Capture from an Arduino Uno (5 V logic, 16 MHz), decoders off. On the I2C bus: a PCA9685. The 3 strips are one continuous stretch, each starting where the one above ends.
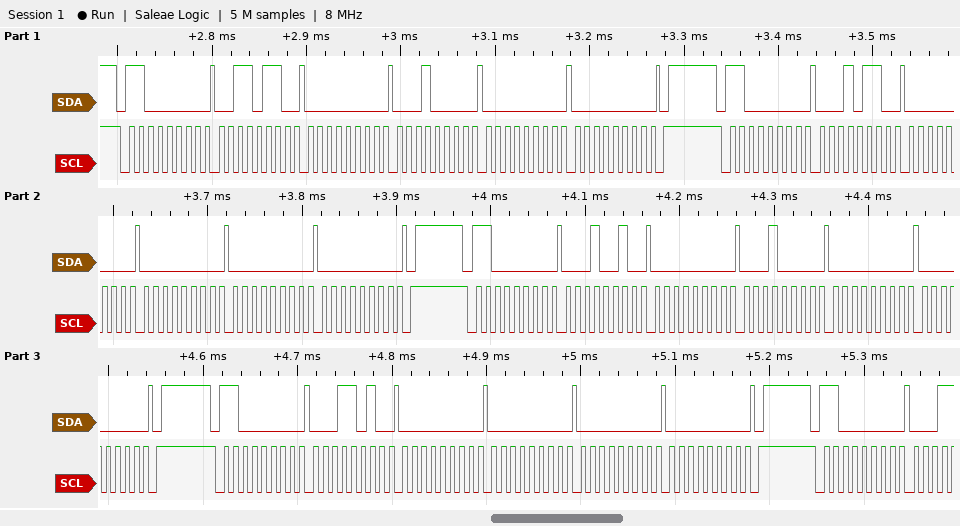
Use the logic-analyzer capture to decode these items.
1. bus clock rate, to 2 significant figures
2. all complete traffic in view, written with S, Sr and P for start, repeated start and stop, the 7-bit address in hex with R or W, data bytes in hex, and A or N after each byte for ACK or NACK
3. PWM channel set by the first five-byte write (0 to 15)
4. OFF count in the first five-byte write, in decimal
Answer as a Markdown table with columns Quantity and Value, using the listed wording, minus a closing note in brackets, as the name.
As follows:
| Quantity | Value |
|---|---|
| bus clock rate, to 2 significant figures | 100 kHz |
| all complete traffic in view, written with S, Sr and P for start, repeated start and stop, the 7-bit address in hex with R or W, data bytes in hex, and A or N after each byte for ACK or NACK | S 60W A 36 A 00 A 10 A 00 A 00 A P S 60W A 16 A 00 A 00 A 00 A 00 A P S 60W A 12 A 00 A 10 A 00 A 00 A P S 60W A 1A A 00 A 00 A 00 A 00 A P S 60W A |
| PWM channel set by the first five-byte write | 12 |
| OFF count in the first five-byte write, in decimal | 0 |
